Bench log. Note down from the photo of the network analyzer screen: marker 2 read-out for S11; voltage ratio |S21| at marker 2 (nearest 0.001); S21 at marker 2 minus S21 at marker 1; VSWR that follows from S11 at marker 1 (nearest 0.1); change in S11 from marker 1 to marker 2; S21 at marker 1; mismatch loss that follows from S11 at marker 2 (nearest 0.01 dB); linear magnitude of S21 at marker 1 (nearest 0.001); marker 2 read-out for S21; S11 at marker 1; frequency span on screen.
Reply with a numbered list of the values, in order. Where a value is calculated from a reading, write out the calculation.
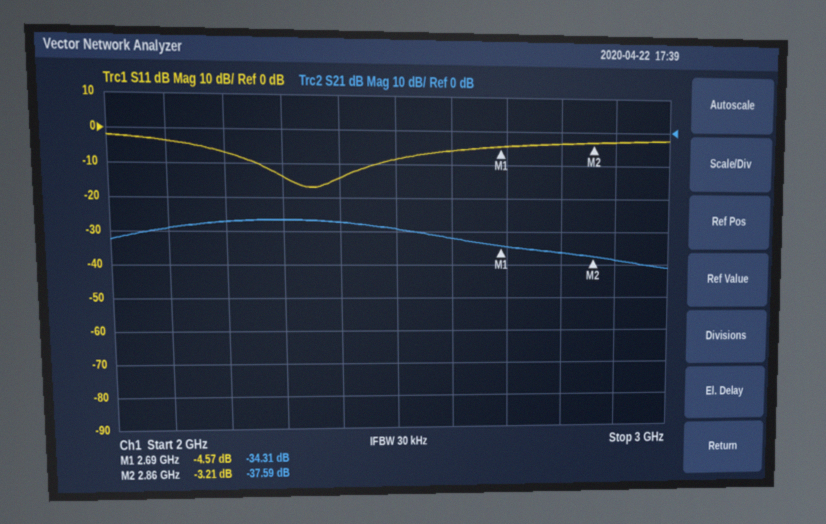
1. -3.21 dB
2. 10^(-37.59/20) ≈ 0.013
3. -37.59 − (-34.31) = -3.28 dB
4. (1 + 0.5909)/(1 − 0.5909) ≈ 3.9
5. -3.21 − (-4.57) = 1.36 dB
6. -34.31 dB
7. −10 log10(1 − 10^(-3.21/10)) ≈ 2.82 dB
8. 10^(-34.31/20) ≈ 0.019
9. -37.59 dB
10. -4.57 dB
11. 1 GHz
